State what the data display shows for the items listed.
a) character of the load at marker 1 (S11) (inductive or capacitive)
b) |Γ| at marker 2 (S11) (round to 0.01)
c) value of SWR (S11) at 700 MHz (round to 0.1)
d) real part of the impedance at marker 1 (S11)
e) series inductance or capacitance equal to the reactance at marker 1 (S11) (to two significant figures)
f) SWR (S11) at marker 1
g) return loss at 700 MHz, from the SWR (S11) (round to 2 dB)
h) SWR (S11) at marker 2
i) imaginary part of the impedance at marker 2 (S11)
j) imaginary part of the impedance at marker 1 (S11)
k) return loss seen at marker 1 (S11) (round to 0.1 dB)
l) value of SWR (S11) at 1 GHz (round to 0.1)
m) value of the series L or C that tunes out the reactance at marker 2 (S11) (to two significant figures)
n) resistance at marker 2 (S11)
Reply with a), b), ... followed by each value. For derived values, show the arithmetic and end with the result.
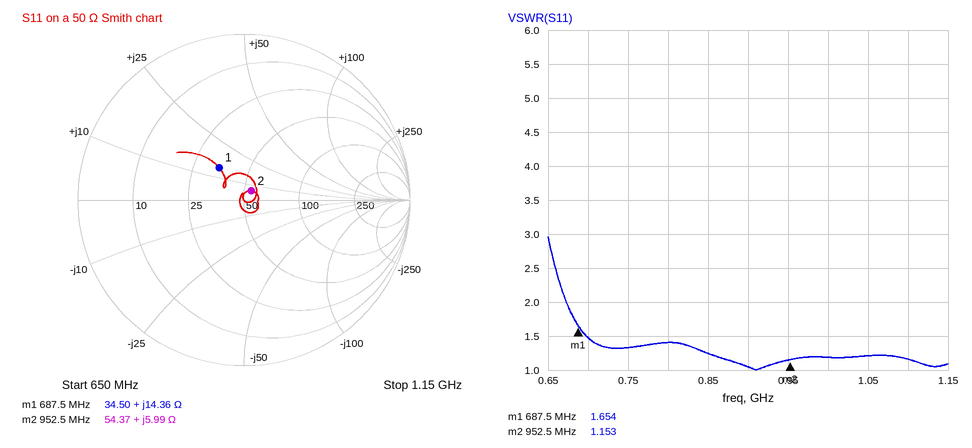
a) inductive
b) 0.07
c) 1.5
d) 34.50 Ω
e) L = 14.36 Ω/(2π × 687.5 MHz) ≈ 3.3 nH
f) 1.654
g) −20 log10((1.5 − 1)/(1.5 + 1)) ≈ 14 dB
h) 1.153
i) +5.99 Ω
j) +14.36 Ω
k) 12.2 dB
l) 1.2
m) C = 1/(2π × 952.5 MHz × 5.99 Ω) ≈ 28 pF
n) 54.37 Ω
